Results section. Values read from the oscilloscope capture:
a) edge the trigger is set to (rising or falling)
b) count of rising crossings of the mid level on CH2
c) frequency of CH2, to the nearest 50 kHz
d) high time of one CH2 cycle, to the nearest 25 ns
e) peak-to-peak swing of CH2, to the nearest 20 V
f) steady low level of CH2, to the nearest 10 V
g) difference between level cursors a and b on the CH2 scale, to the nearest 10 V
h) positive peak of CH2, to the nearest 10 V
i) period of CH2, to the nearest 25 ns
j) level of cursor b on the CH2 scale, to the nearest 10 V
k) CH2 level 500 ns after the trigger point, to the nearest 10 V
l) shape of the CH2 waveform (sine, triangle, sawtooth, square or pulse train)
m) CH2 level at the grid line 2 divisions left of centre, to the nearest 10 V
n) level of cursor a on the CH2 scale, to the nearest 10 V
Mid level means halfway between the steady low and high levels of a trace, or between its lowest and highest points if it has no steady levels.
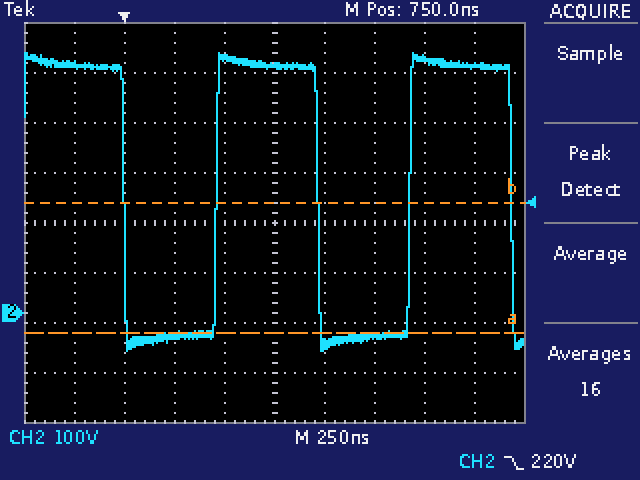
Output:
falling
2
1.05 MHz
500 ns
600 V
-50 V
260 V
520 V
975 ns
220 V
510 V
square
-50 V
-40 V
